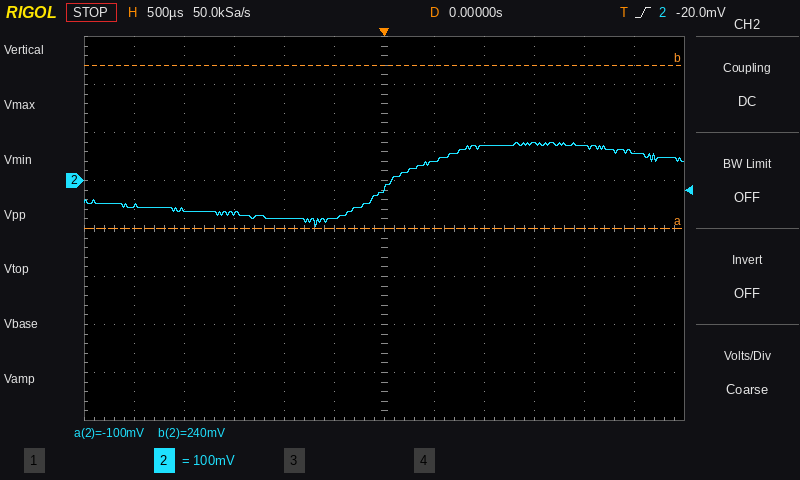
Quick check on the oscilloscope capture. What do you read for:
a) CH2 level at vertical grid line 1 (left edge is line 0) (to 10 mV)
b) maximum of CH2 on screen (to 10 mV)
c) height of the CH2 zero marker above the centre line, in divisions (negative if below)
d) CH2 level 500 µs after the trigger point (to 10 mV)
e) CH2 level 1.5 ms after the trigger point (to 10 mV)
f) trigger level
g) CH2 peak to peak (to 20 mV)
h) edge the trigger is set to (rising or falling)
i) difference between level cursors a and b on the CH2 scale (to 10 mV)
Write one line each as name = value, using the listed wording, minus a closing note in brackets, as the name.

CH2 level at vertical grid line 1 (left edge is line 0) = -50 mV
maximum of CH2 on screen = 80 mV
height of the CH2 zero marker above the centre line, in divisions = +1.0 div
CH2 level 500 µs after the trigger point = 40 mV
CH2 level 1.5 ms after the trigger point = 80 mV
trigger level = -20.0 mV
CH2 peak to peak = 180 mV
edge the trigger is set to = rising
difference between level cursors a and b on the CH2 scale = 340 mV
